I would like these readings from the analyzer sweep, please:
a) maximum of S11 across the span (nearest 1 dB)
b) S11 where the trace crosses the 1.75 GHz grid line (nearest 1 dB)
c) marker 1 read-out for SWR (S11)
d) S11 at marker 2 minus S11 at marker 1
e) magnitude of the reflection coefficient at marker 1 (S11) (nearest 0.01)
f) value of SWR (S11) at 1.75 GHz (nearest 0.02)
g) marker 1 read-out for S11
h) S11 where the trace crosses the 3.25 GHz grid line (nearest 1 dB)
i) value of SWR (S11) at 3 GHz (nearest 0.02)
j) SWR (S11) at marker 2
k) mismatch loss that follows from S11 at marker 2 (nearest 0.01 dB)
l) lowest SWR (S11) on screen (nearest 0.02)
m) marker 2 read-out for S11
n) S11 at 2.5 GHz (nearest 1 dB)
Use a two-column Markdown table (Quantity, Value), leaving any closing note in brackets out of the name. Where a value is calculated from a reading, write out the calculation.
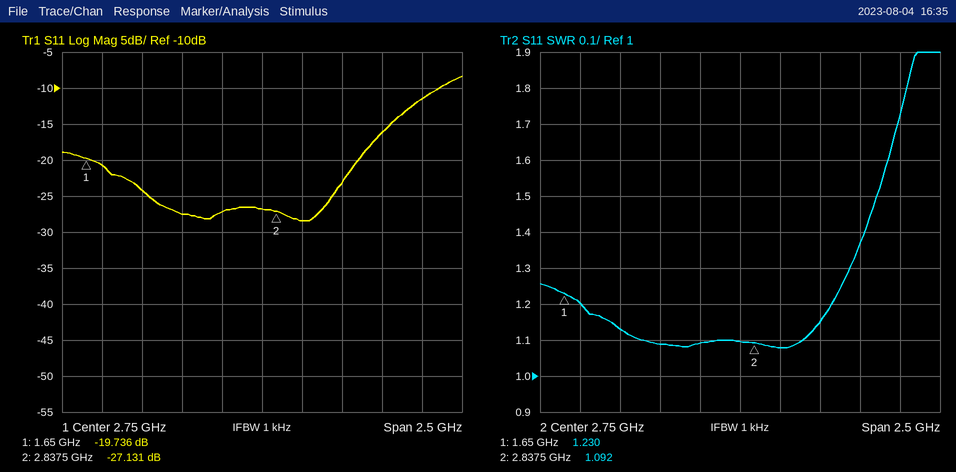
| Quantity | Value |
|---|---|
| maximum of S11 across the span | -8 dB |
| S11 where the trace crosses the 1.75 GHz grid line | -21 dB |
| marker 1 read-out for SWR | 1.230 |
| S11 at marker 2 minus S11 at marker 1 | -27.131 − (-19.736) = -7.395 dB |
| magnitude of the reflection coefficient at marker 1 (S11) | 10^(-19.736/20) ≈ 0.10 |
| value of SWR (S11) at 1.75 GHz | 1.20 |
| marker 1 read-out for S11 | -19.736 dB |
| S11 where the trace crosses the 3.25 GHz grid line | -23 dB |
| value of SWR (S11) at 3 GHz | 1.08 |
| SWR (S11) at marker 2 | 1.092 |
| mismatch loss that follows from S11 at marker 2 | −10 log10(1 − 10^(-27.131/10)) ≈ 0.01 dB |
| lowest SWR (S11) on screen | 1.08 |
| marker 2 read-out for S11 | -27.131 dB |
| S11 at 2.5 GHz | -27 dB |
